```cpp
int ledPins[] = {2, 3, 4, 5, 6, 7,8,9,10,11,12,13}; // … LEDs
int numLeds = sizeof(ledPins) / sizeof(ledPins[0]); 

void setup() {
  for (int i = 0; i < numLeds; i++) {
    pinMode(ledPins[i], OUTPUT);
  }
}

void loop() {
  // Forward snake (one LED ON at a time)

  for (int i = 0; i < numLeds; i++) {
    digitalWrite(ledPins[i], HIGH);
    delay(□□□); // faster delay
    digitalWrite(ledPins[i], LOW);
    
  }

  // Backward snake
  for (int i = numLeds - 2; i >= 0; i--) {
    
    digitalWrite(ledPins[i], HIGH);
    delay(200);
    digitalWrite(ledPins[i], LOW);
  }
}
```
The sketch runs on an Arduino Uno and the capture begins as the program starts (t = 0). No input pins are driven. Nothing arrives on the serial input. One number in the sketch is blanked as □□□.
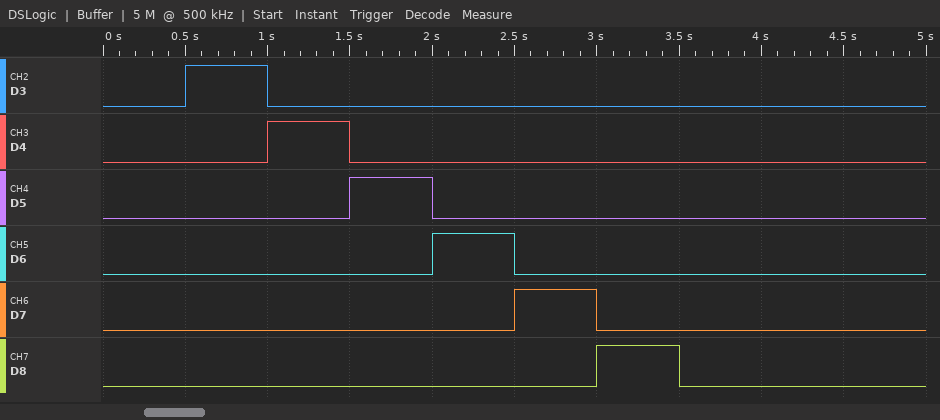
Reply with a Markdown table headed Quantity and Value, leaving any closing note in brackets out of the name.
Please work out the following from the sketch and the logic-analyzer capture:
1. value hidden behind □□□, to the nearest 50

| Quantity | Value |
|---|---|
| value hidden behind □□□, to the nearest 50 | 500 |
